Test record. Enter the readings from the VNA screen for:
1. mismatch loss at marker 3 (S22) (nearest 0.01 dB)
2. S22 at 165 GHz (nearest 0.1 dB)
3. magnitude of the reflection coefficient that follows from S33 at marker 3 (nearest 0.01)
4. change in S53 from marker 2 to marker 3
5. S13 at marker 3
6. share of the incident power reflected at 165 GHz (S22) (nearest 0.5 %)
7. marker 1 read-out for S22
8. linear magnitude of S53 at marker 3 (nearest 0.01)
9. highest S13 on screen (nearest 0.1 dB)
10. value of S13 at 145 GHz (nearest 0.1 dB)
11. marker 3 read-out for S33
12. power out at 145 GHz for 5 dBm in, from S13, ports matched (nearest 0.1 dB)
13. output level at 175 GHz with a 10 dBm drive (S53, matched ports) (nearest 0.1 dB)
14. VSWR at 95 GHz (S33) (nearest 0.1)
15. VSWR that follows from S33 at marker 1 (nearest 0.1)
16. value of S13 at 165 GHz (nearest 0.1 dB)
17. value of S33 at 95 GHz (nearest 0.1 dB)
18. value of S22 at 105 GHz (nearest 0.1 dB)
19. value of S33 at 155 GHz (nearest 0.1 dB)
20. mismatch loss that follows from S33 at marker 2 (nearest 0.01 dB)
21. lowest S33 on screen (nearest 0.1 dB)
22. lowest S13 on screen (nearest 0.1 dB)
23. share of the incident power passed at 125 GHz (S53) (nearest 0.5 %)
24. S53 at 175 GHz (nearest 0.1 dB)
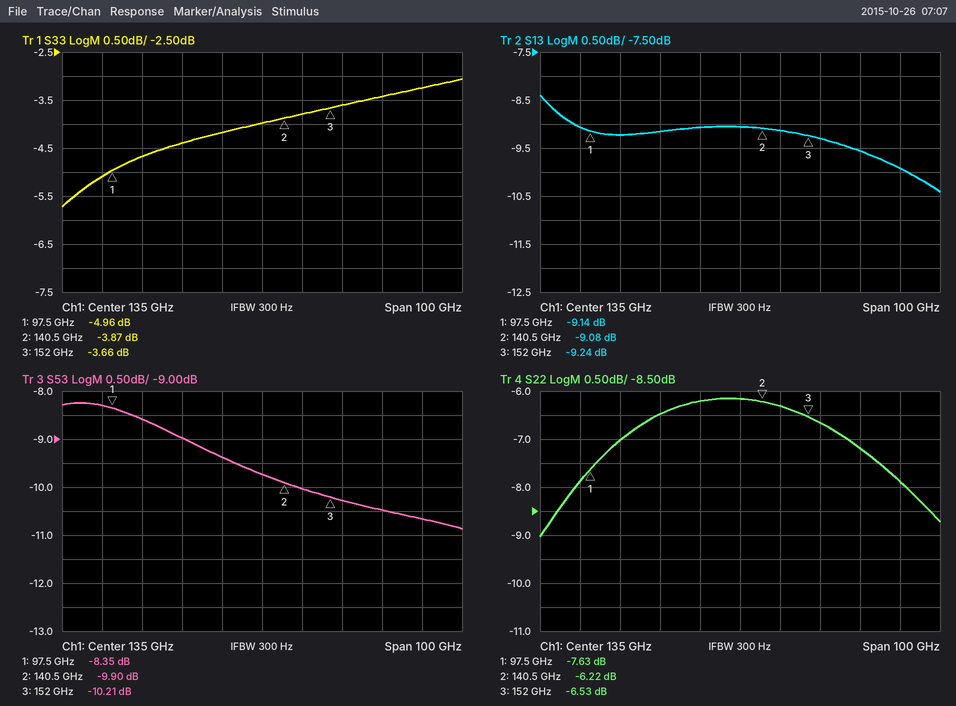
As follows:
1.09 dB
-7.2 dB
0.66
-0.31 dB
-9.24 dB
19.0 %
-7.63 dB
0.31
-8.4 dB
-9.1 dB
-3.66 dB
-4.1 dBm
-0.7 dBm
3.5
3.6
-9.6 dB
-5.1 dB
-7.0 dB
-3.6 dB
2.29 dB
-5.7 dB
-10.4 dB
11.5 %
-10.7 dB
